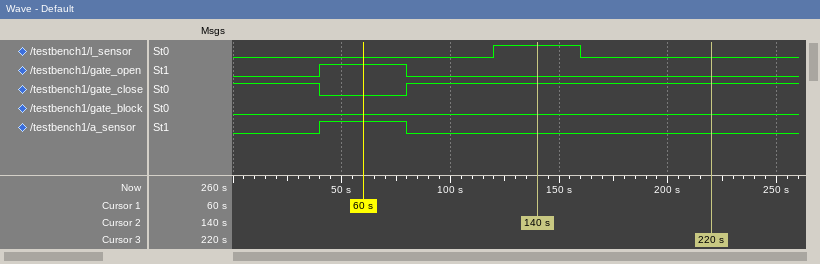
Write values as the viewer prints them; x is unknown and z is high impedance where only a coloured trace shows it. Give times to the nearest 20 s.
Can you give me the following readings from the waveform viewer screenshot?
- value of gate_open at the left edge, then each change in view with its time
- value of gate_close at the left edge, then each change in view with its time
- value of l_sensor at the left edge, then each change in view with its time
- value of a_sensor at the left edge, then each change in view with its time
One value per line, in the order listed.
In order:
0, 1 at 40 s, 0 at 80 s
1, 0 at 40 s, 1 at 80 s
0, 1 at 120 s, 0 at 160 s
0, 1 at 40 s, 0 at 80 s
